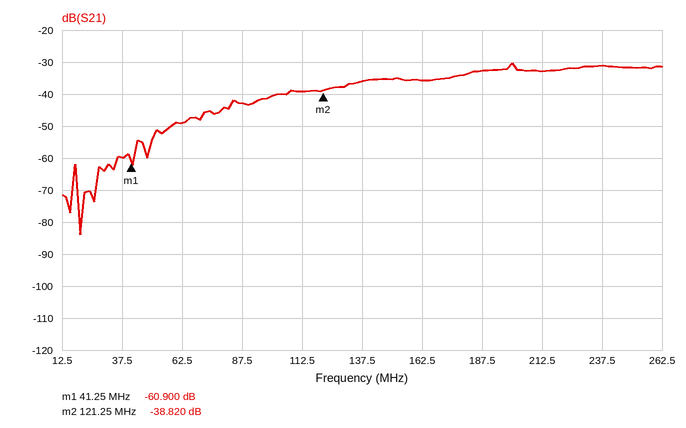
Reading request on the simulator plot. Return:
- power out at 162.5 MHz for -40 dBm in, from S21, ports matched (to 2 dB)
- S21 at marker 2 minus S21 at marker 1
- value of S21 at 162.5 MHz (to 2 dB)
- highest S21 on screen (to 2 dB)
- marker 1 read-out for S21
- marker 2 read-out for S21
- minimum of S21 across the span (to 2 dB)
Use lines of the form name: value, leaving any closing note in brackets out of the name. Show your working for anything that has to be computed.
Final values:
power out at 162.5 MHz for -40 dBm in, from S21, ports matched: -40 dBm + (-36 dB) = -76 dBm
S21 at marker 2 minus S21 at marker 1: -38.82 − (-60.9) = 22.080 dB
value of S21 at 162.5 MHz: -36 dB
highest S21 on screen: -30 dB
marker 1 read-out for S21: -60.900 dB
marker 2 read-out for S21: -38.820 dB
minimum of S21 across the span: -84 dB
